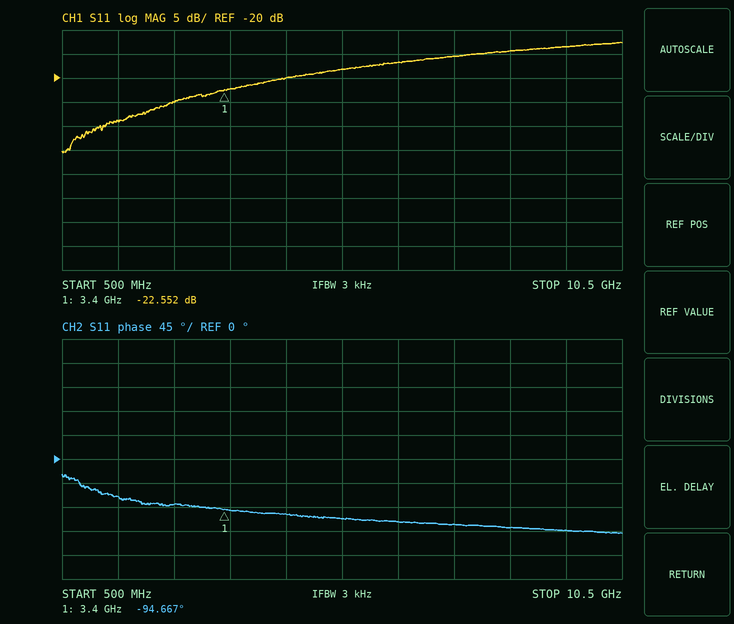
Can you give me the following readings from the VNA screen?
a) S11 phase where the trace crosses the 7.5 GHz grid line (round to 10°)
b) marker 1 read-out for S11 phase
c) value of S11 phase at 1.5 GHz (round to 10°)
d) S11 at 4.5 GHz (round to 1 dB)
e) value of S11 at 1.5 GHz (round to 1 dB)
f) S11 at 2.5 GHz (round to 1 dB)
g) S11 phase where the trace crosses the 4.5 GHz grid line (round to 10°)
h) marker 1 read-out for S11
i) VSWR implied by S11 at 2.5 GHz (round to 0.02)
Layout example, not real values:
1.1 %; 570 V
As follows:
-120°; -94.667°; -70°; -20 dB; -29 dB; -25 dB; -100°; -22.552 dB; 1.12
